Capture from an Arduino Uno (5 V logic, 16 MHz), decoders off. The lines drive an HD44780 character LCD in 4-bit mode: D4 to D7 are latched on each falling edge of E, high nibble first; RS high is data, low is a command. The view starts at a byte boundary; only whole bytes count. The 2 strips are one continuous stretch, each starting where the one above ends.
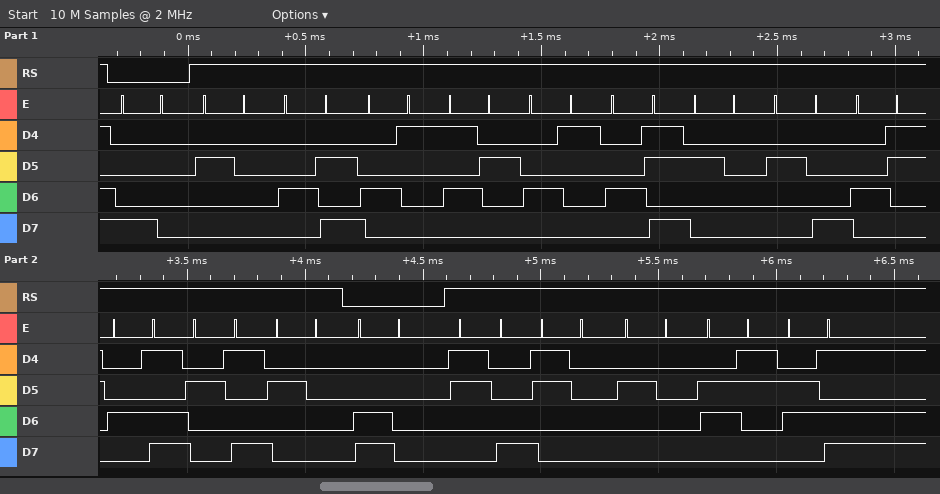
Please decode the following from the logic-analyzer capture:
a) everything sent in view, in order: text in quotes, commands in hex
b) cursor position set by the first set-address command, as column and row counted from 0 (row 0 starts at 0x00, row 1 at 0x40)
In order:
0x80 " JARAK (CM) " 0xC0 "80 cm"
column 0, row 0
